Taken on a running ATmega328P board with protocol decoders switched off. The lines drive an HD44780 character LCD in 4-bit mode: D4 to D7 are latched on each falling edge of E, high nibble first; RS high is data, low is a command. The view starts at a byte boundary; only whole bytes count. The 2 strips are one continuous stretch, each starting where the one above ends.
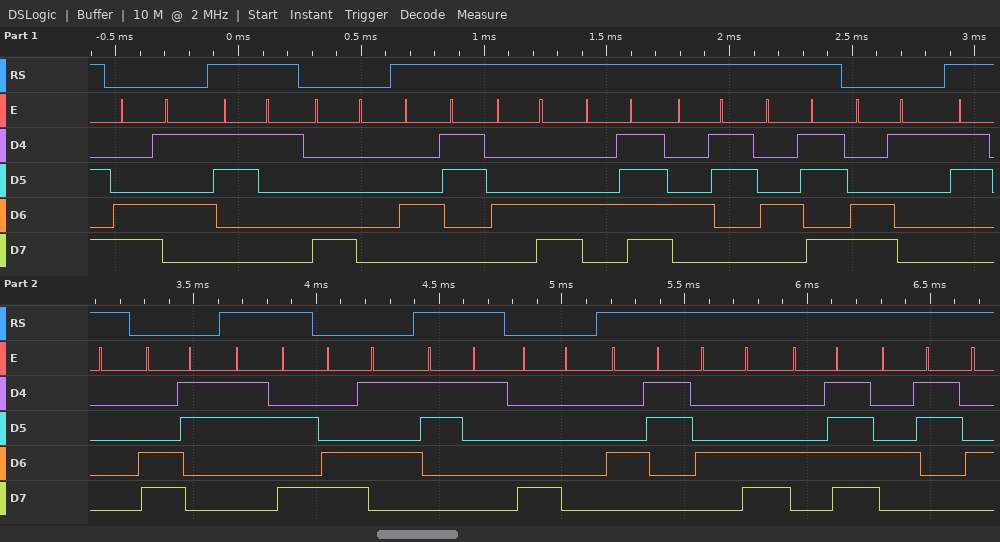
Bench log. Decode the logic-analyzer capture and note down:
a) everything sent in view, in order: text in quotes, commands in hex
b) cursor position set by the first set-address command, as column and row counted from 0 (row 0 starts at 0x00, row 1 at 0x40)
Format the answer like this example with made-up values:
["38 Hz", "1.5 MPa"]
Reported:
["0xC5 \"1\" 0x80 \"CLOCK\" 0xC1 \"0\" 0xC3 \":\" 0xC5 \"1\" 0x80 \"CLOC\"", "column 5, row 1"]
